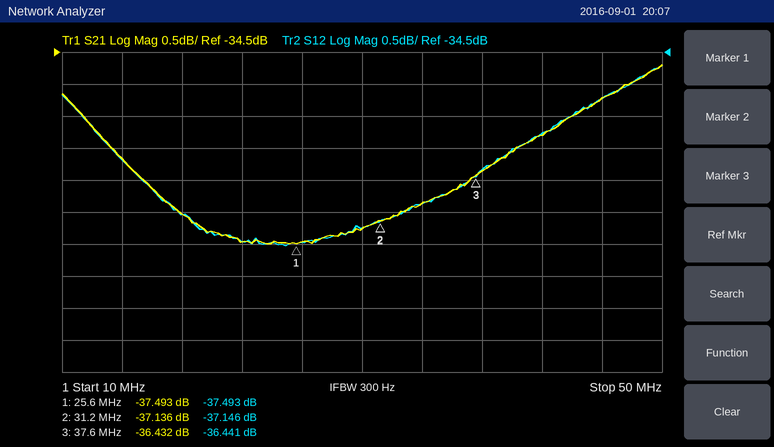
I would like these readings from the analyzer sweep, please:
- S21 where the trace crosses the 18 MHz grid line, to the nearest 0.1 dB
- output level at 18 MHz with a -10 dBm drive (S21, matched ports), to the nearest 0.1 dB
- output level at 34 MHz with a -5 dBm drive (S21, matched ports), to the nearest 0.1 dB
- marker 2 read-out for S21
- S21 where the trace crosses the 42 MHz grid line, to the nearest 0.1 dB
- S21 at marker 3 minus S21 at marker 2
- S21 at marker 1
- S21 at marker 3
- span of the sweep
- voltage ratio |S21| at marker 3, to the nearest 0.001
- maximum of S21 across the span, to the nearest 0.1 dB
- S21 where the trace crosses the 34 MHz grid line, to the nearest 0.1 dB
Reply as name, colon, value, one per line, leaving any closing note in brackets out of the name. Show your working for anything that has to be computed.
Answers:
S21 where the trace crosses the 18 MHz grid line, to the nearest 0.1 dB: -37.0 dB
output level at 18 MHz with a -10 dBm drive (S21, matched ports), to the nearest 0.1 dB: -10 dBm + (-37.0 dB) = -47.0 dBm
output level at 34 MHz with a -5 dBm drive (S21, matched ports), to the nearest 0.1 dB: -5 dBm + (-36.9 dB) = -41.9 dBm
marker 2 read-out for S21: -37.136 dB
S21 where the trace crosses the 42 MHz grid line, to the nearest 0.1 dB: -35.8 dB
S21 at marker 3 minus S21 at marker 2: -36.432 − (-37.136) = 0.704 dB
S21 at marker 1: -37.493 dB
S21 at marker 3: -36.432 dB
span of the sweep: 40 MHz
voltage ratio |S21| at marker 3, to the nearest 0.001: 10^(-36.432/20) ≈ 0.015
maximum of S21 across the span, to the nearest 0.1 dB: -34.7 dB
S21 where the trace crosses the 34 MHz grid line, to the nearest 0.1 dB: -36.9 dB
